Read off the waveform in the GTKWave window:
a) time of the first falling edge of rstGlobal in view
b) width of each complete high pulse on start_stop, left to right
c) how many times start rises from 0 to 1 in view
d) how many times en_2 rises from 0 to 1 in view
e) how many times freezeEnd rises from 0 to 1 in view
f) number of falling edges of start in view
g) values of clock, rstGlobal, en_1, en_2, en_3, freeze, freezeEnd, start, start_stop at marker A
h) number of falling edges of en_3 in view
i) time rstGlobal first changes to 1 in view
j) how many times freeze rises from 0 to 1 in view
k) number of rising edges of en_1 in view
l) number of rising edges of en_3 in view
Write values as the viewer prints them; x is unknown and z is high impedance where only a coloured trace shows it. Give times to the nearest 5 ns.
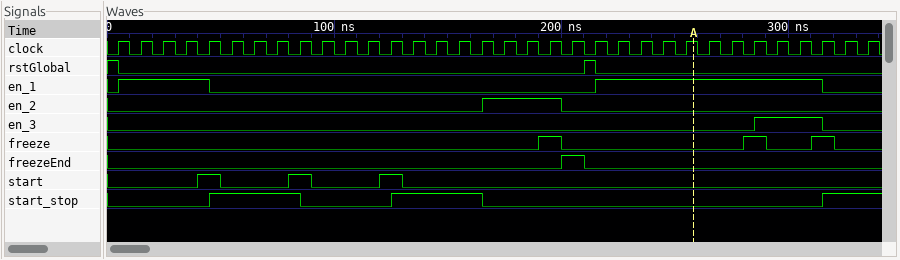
5 ns
40 ns, 40 ns
3
1
1
3
clock=1, rstGlobal=0, en_1=1, en_2=0, en_3=0, freeze=0, freezeEnd=0, start=0, start_stop=0
1
210 ns
3
2
1
